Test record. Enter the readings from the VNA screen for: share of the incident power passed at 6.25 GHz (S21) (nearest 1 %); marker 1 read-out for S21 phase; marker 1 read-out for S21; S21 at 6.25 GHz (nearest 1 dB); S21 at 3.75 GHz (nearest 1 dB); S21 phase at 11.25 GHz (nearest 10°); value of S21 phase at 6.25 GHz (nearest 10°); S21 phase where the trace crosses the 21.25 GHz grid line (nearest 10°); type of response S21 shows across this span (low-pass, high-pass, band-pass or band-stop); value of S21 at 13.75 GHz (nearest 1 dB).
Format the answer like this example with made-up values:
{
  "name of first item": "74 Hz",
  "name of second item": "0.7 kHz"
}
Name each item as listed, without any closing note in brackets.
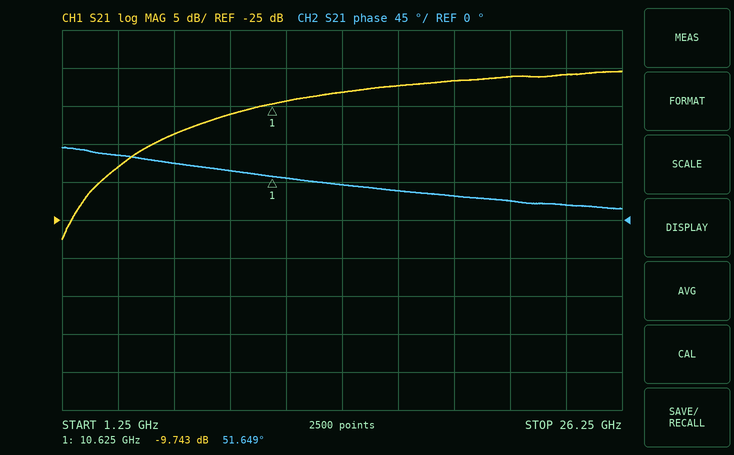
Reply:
{
  "share of the incident power passed at 6.25 GHz (S21)": "4 %",
  "marker 1 read-out for S21 phase": "51.649°",
  "marker 1 read-out for S21": "-9.743 dB",
  "S21 at 6.25 GHz": "-14 dB",
  "S21 at 3.75 GHz": "-18 dB",
  "S21 phase at 11.25 GHz": "50°",
  "value of S21 phase at 6.25 GHz": "70°",
  "S21 phase where the trace crosses the 21.25 GHz grid line": "20°",
  "type of response S21 shows across this span": "high-pass",
  "value of S21 at 13.75 GHz": "-8 dB"
}
